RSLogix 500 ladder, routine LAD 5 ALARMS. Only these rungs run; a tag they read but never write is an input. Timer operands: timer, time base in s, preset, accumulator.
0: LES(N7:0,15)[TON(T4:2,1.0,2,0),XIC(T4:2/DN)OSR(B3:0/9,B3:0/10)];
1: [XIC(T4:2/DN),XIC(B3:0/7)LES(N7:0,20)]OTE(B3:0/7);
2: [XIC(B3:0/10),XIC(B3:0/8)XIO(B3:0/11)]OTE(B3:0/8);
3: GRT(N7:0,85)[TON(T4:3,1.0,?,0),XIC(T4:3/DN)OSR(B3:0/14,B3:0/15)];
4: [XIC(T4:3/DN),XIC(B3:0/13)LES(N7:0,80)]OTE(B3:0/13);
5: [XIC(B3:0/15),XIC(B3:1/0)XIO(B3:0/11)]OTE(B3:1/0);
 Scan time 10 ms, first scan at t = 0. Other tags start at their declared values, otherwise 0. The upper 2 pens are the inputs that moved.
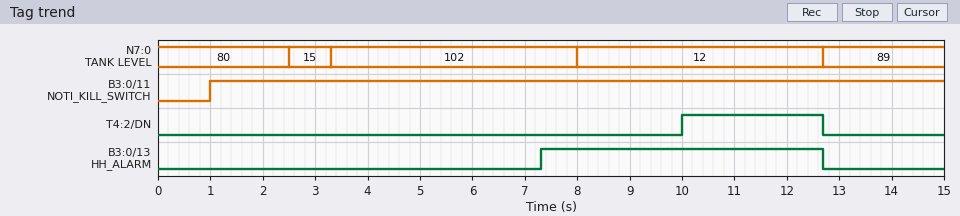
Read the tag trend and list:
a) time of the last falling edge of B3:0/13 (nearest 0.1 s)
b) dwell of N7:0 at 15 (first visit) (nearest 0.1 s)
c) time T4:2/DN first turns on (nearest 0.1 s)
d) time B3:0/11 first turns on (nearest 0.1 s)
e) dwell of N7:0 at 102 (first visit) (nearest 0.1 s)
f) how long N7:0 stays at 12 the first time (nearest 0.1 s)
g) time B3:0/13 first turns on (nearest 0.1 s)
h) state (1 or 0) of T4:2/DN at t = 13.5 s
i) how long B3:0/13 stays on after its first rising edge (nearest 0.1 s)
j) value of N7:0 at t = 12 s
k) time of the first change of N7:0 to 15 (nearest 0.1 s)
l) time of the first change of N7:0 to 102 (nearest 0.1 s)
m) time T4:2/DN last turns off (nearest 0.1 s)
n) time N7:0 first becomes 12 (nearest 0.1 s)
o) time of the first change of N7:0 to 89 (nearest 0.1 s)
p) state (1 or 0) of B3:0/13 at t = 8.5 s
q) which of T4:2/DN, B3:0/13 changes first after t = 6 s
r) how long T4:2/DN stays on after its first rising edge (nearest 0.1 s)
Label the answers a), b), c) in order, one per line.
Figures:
a) 12.7 s
b) 0.8 s
c) 10.0 s
d) 1.0 s
e) 4.7 s
f) 4.7 s
g) 7.3 s
h) 0
i) 5.4 s
j) 12
k) 2.5 s
l) 3.3 s
m) 12.7 s
n) 8.0 s
o) 12.7 s
p) 1
q) B3:0/13
r) 2.7 s
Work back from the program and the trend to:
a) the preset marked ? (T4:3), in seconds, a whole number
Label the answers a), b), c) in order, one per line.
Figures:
a) 4 s
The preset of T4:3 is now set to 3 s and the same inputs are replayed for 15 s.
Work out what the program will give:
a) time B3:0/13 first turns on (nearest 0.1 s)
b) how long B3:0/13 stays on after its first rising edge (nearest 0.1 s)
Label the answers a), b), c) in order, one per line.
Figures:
a) 6.3 s
b) 6.4 s
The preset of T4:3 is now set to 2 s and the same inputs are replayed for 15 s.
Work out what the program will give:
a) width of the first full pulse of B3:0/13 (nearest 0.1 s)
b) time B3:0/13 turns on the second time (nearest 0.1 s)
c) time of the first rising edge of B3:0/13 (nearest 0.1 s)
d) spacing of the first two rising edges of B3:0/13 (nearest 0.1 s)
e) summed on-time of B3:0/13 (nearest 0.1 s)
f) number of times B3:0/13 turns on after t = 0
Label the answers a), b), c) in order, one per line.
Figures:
a) 7.4 s
b) 14.7 s
c) 5.3 s
d) 9.4 s
e) 7.7 s
f) 2
